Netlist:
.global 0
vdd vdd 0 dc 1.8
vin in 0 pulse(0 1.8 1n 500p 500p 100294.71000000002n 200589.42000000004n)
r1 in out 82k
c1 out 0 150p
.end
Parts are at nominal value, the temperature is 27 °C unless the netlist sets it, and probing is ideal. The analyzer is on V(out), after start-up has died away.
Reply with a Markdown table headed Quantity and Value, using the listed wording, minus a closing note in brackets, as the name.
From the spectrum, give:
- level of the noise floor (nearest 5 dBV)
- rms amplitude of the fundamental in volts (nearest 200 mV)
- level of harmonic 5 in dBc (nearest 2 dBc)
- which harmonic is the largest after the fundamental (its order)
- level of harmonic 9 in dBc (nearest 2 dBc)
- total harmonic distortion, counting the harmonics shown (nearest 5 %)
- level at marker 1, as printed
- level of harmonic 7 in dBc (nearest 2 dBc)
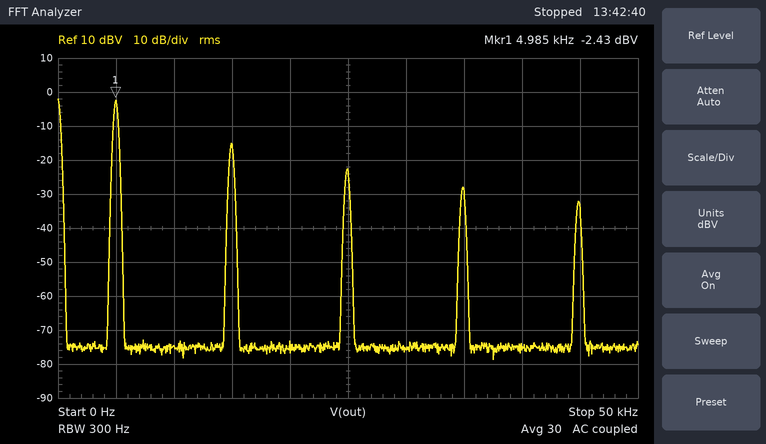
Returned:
| Quantity | Value |
|---|---|
| level of the noise floor | -75 dBV |
| rms amplitude of the fundamental in volts | 800 mV |
| level of harmonic 5 in dBc | -20 dBc |
| which harmonic is the largest after the fundamental | 3 |
| level of harmonic 9 in dBc | -30 dBc |
| total harmonic distortion, counting the harmonics shown | 25 % |
| level at marker 1, as printed | -2.43 dBV |
| level of harmonic 7 in dBc | -26 dBc |
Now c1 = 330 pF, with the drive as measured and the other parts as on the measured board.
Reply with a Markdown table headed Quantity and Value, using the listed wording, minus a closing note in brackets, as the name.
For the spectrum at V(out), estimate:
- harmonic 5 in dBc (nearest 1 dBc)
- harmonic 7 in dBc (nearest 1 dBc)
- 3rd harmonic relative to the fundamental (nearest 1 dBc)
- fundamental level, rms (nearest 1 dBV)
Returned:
| Quantity | Value |
|---|---|
| harmonic 5 in dBc | -24 dBc |
| harmonic 7 in dBc | -30 dBc |
| 3rd harmonic relative to the fundamental | -16 dBc |
| fundamental level, rms | -4 dBV |
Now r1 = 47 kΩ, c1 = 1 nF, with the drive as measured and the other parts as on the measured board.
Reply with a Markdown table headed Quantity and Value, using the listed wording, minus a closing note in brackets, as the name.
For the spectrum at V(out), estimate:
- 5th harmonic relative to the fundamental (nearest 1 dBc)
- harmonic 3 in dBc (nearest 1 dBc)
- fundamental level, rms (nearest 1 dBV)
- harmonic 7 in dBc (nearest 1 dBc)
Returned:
| Quantity | Value |
|---|---|
| 5th harmonic relative to the fundamental | -26 dBc |
| harmonic 3 in dBc | -18 dBc |
| fundamental level, rms | -7 dBV |
| harmonic 7 in dBc | -32 dBc |
